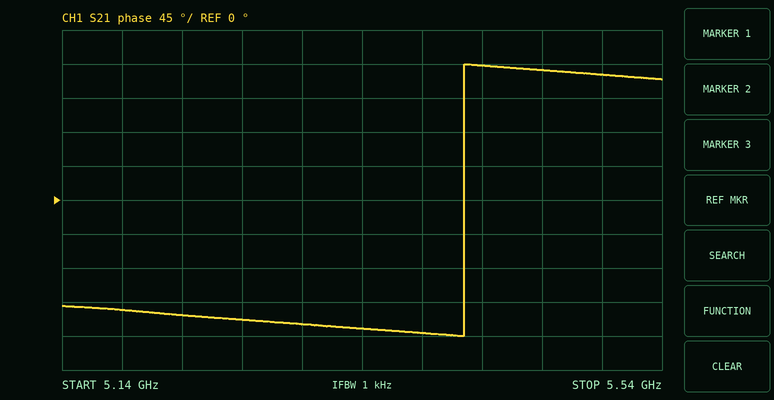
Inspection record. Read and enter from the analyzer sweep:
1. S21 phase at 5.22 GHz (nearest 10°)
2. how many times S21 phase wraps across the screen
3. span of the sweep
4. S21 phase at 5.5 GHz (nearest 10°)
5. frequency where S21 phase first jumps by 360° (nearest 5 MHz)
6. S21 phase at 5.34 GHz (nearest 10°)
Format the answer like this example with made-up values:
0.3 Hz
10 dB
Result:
-150°
1
400 MHz
170°
5.410 GHz
-170°
